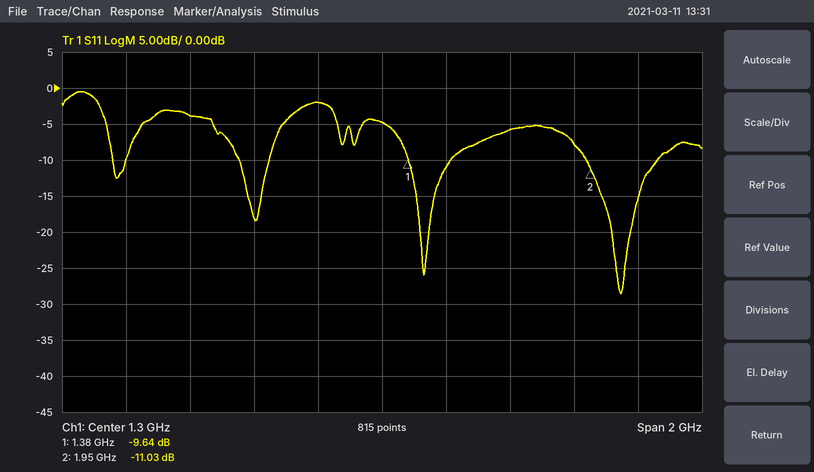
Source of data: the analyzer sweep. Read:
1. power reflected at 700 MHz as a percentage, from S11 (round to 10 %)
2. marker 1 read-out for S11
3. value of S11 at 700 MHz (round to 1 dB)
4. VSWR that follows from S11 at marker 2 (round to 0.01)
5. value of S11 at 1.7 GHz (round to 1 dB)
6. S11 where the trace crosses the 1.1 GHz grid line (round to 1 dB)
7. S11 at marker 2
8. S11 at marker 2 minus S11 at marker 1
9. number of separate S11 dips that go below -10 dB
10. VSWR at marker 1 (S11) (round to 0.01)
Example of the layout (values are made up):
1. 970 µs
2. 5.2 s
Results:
1. 40 %
2. -9.64 dB
3. -4 dB
4. 1.78
5. -6 dB
6. -2 dB
7. -11.03 dB
8. -1.39 dB
9. 4
10. 1.98
